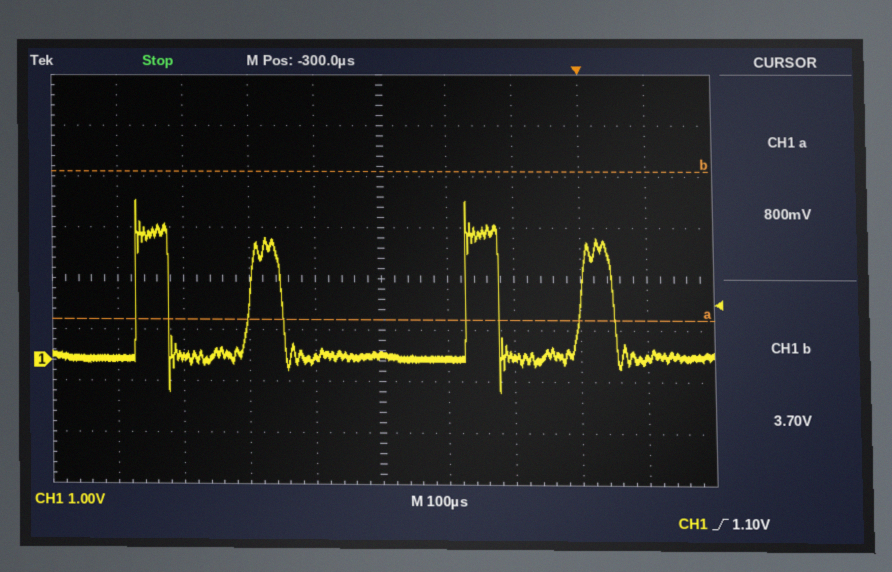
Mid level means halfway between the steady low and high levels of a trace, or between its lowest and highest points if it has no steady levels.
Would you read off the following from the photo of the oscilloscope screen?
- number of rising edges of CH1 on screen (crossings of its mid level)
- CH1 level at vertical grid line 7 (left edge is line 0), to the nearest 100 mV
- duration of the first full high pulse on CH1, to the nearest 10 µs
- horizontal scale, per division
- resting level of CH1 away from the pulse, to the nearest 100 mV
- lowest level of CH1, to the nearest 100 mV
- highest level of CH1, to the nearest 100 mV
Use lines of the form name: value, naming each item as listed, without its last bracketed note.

number of rising edges of CH1 on screen: 4
CH1 level at vertical grid line 7 (left edge is line 0), to the nearest 100 mV: 100 mV
duration of the first full high pulse on CH1, to the nearest 10 µs: 50 µs
horizontal scale, per division: 100 µs
resting level of CH1 away from the pulse, to the nearest 100 mV: 100 mV
lowest level of CH1, to the nearest 100 mV: -600 mV
highest level of CH1, to the nearest 100 mV: 3.1 V
